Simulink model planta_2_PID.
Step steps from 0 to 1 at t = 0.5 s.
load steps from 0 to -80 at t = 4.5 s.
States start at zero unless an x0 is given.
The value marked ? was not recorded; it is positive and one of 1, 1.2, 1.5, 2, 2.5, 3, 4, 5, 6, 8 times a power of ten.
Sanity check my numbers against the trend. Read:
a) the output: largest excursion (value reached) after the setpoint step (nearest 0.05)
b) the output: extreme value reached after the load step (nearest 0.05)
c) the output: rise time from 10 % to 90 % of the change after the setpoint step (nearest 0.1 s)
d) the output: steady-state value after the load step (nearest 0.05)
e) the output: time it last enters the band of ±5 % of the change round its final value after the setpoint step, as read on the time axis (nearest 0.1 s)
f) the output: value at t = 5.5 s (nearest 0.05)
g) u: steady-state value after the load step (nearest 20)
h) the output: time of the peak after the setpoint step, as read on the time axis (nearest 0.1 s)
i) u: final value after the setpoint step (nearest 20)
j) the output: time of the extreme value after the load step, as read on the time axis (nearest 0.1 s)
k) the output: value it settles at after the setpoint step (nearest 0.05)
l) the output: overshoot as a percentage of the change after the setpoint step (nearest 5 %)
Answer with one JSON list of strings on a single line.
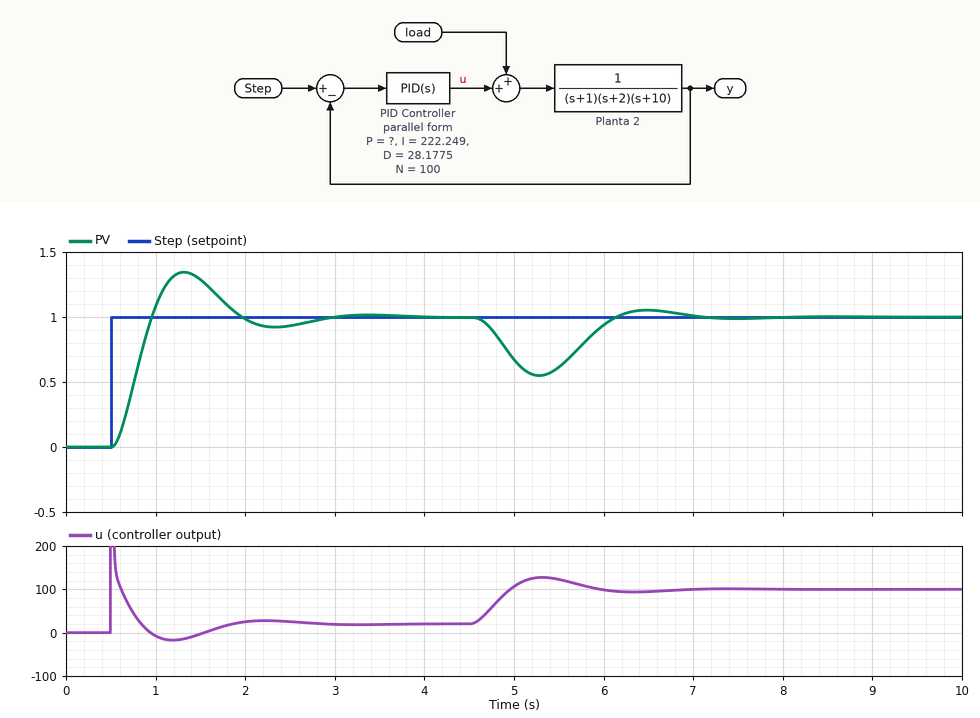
["1.35", "0.55", "0.3 s", "1.00", "2.6 s", "0.60", "100", "1.3 s", "20", "5.3 s", "1.00", "35 %"]
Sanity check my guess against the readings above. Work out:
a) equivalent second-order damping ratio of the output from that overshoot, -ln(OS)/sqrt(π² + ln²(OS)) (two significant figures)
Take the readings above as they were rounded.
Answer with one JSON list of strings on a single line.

["0.32"]
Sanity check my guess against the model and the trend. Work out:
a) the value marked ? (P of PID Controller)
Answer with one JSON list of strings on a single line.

["150"]
